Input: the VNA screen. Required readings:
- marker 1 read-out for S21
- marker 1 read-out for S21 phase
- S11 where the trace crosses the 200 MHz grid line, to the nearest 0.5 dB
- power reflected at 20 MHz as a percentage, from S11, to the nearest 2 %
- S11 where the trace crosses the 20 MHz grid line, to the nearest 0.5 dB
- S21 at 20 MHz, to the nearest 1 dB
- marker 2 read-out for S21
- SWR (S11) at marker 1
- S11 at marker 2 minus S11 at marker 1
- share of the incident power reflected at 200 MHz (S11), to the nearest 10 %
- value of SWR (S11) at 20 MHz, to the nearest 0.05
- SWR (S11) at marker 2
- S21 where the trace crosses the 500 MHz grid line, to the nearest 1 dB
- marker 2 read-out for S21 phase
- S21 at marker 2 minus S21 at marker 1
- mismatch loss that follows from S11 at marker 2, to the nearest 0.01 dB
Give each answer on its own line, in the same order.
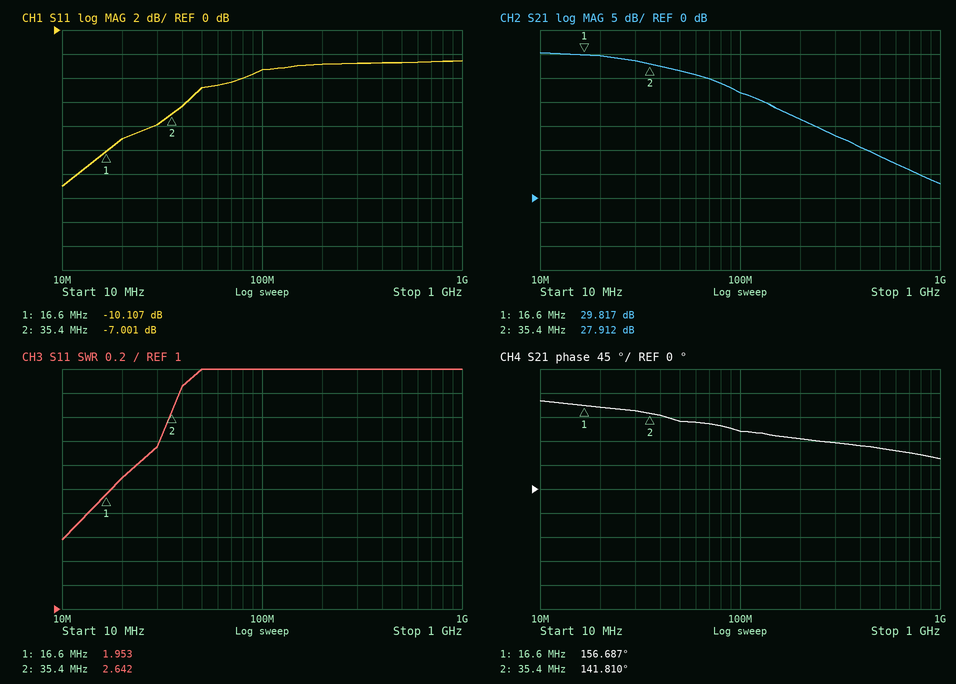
29.817 dB
156.687°
-3.0 dB
12 %
-9.0 dB
30 dB
27.912 dB
1.953
3.106 dB
50 %
2.10
2.642
9 dB
141.810°
-1.905 dB
0.97 dB
